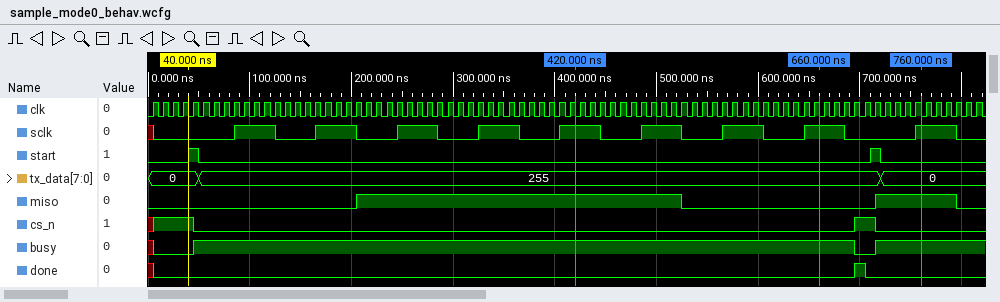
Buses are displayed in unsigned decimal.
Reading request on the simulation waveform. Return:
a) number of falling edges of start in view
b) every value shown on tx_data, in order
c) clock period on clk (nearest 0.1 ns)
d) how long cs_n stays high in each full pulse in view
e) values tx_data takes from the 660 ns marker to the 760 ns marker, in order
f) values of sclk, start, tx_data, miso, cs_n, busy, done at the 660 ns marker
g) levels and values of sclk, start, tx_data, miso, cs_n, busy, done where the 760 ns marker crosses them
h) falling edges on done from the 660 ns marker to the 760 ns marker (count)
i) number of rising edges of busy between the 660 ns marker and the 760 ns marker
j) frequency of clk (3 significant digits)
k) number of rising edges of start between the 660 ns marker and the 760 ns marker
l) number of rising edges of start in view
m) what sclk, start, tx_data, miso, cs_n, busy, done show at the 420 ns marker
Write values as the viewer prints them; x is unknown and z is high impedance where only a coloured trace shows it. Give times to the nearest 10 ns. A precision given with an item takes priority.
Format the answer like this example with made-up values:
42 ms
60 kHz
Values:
2
0, 255, 0
10 ns
20 ns
255, 0
sclk=1, start=0, tx_data=255, miso=0, cs_n=0, busy=1, done=0
sclk=1, start=0, tx_data=0, miso=1, cs_n=0, busy=1, done=0
1
1
100 MHz
1
2
sclk=1, start=0, tx_data=255, miso=1, cs_n=0, busy=1, done=0
